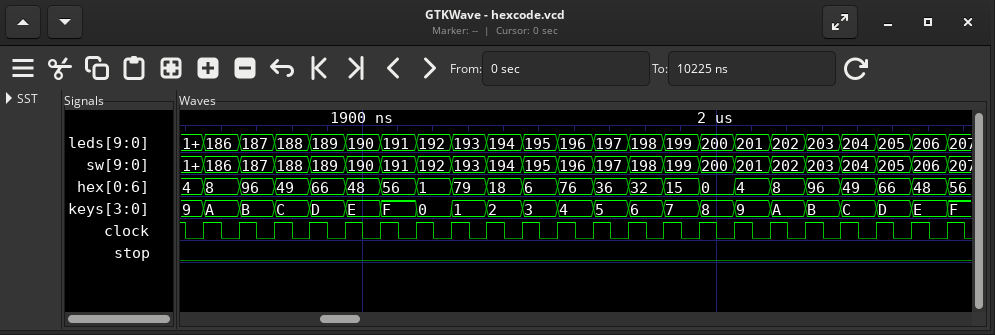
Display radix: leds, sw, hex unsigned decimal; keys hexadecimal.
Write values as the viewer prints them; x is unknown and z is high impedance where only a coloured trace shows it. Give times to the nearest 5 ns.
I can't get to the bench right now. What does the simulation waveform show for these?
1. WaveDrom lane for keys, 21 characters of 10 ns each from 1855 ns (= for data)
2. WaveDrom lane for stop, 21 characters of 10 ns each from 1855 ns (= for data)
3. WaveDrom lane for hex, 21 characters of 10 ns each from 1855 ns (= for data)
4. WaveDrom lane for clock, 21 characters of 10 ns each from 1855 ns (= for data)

{name: 'keys', wave: '=====================', data: 'A B C D E F 0 1 2 3 4 5 6 7 8 9 A B C D E'}
{name: 'stop', wave: '0....................'}
{name: 'hex', wave: '=====================', data: '8 96 49 66 48 56 1 79 18 6 76 36 32 15 0 4 8 96 49 66 48'}
{name: 'clock', wave: 'p....................'}
